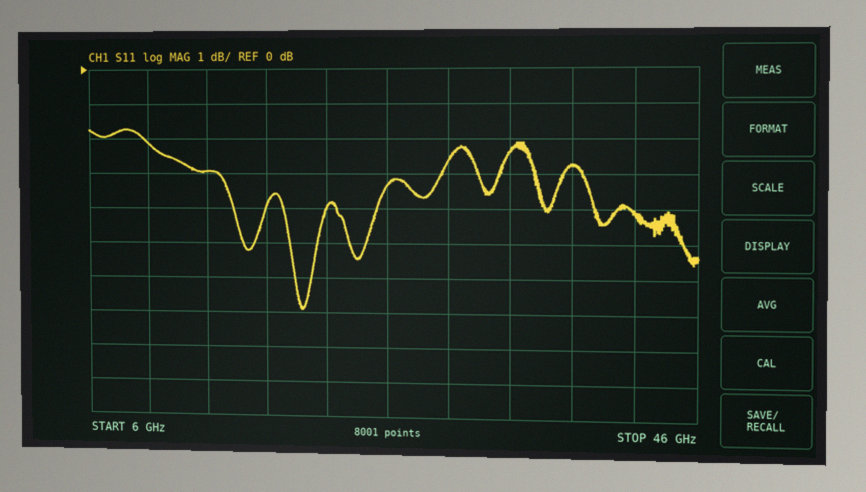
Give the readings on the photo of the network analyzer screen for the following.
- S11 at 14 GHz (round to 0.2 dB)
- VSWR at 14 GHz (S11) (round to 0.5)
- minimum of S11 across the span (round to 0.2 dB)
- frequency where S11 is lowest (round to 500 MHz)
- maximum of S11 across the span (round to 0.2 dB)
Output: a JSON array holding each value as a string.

["-3.0 dB", "6.0", "-7.0 dB", "20.5 GHz", "-1.8 dB"]
